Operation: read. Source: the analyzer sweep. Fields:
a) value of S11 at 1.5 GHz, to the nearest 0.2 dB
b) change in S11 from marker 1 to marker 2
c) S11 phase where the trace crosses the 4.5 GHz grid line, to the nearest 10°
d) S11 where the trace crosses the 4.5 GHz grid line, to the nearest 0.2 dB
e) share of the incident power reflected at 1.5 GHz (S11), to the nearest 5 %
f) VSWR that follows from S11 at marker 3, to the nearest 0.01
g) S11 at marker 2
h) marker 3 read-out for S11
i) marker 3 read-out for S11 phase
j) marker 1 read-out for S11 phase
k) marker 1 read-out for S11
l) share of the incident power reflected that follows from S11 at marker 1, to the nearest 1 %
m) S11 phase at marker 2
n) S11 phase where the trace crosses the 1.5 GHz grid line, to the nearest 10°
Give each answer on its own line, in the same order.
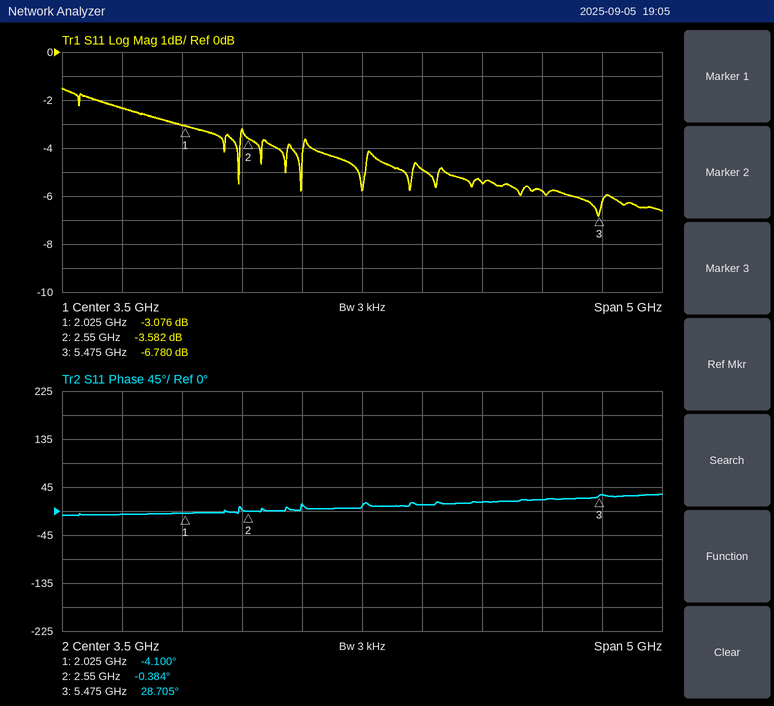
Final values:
-2.4 dB
-0.506 dB
20°
-5.4 dB
60 %
2.69
-3.582 dB
-6.780 dB
28.705°
-4.100°
-3.076 dB
49 %
-0.384°
-10°
